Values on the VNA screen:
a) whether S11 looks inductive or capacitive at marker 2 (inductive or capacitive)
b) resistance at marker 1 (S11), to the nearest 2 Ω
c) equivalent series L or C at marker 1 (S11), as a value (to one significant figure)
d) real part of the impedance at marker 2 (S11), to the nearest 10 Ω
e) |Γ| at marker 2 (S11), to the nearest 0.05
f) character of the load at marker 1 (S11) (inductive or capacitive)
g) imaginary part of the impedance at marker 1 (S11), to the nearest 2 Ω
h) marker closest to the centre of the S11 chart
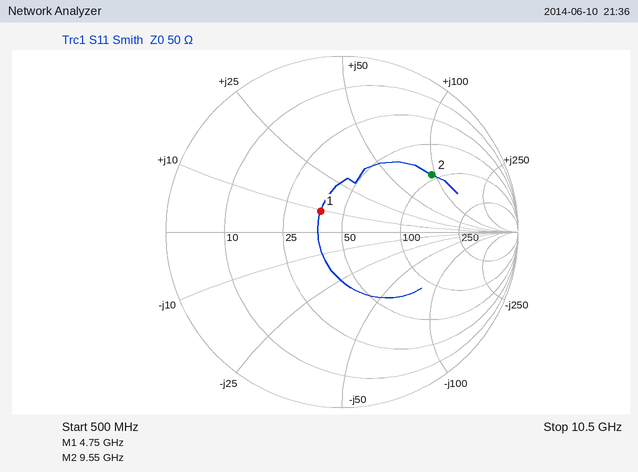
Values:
inductive
38 Ω
300 pH
90 Ω
0.60
inductive
+10 Ω
marker 1
